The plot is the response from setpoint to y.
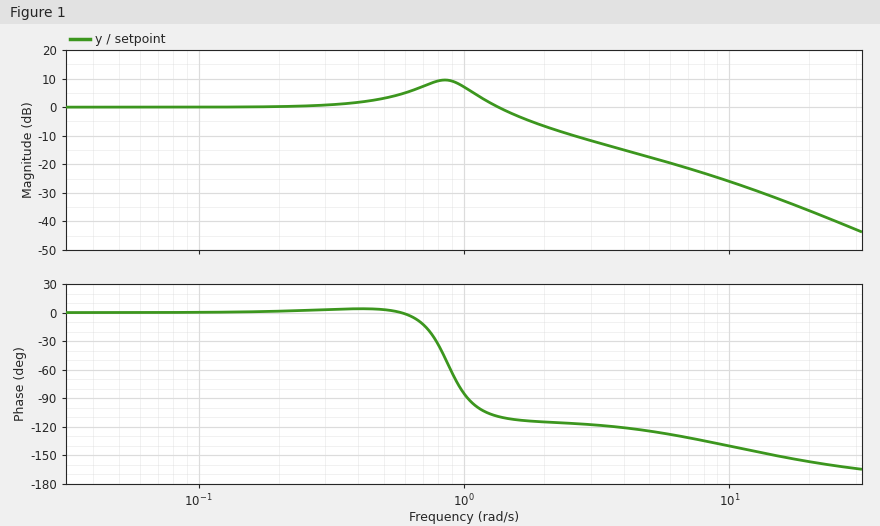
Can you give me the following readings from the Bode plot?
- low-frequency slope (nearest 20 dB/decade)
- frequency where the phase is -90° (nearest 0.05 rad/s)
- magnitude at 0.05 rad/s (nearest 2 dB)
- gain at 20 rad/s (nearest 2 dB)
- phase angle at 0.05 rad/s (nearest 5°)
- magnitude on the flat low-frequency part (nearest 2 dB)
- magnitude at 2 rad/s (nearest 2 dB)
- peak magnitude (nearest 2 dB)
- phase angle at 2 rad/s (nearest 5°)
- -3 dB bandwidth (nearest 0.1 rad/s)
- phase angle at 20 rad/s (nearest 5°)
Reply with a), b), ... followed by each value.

a) 0 dB/decade
b) 1.05 rad/s
c) 0 dB
d) -36 dB
e) 0°
f) 0 dB
g) -6 dB
h) 10 dB
i) -115°
j) 1.6 rad/s
k) -155°
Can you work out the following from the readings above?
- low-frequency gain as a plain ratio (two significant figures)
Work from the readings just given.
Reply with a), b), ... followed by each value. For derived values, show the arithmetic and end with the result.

a) 10^(0 / 20) = 1.0
